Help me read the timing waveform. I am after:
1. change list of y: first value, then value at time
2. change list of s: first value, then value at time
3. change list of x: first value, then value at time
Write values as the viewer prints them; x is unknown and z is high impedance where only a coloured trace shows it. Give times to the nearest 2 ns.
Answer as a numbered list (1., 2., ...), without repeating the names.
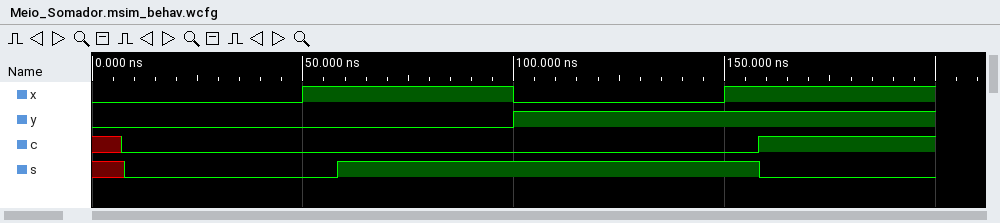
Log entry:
1. 0, 1 at 100 ns
2. x, 0 at 8 ns, 1 at 58 ns, 0 at 158 ns
3. 0, 1 at 50 ns, 0 at 100 ns, 1 at 150 ns
